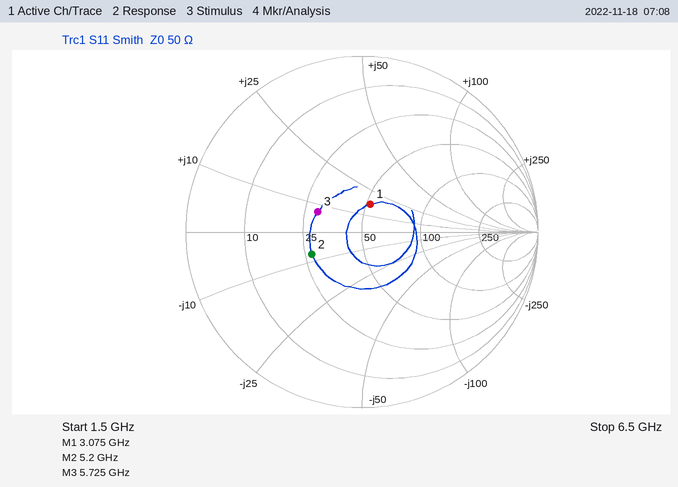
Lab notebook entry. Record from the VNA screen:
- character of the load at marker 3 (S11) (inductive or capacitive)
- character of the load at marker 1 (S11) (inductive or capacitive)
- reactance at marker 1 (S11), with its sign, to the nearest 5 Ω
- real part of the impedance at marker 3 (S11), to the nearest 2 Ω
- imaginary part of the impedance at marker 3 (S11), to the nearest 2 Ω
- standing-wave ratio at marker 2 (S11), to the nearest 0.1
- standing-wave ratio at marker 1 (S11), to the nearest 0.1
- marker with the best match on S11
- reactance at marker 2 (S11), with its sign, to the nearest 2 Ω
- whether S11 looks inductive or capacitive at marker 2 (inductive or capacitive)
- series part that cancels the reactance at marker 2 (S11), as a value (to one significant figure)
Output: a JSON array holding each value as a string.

["inductive", "inductive", "+15 Ω", "30 Ω", "+8 Ω", "1.9", "1.4", "marker 1", "-8 Ω", "capacitive", "200 pH"]
